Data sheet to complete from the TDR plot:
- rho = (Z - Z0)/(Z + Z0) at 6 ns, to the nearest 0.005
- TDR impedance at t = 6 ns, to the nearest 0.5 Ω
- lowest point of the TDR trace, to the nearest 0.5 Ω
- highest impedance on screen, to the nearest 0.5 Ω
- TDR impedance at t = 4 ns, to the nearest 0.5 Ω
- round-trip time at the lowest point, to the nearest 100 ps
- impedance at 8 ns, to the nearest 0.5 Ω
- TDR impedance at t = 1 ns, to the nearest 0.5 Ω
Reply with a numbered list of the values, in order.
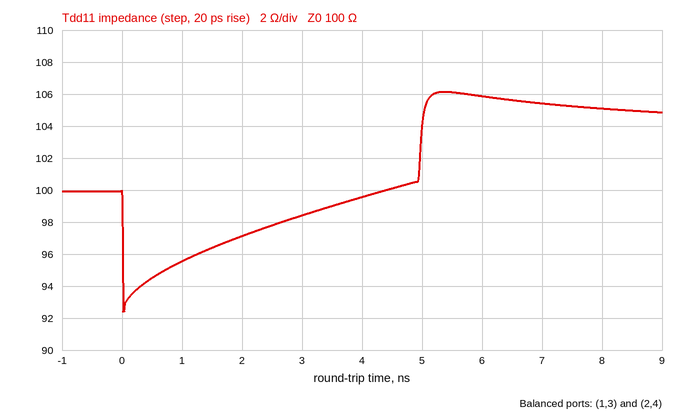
1. +0.030
2. 106.0 Ω
3. 92.5 Ω
4. 106.0 Ω
5. 99.5 Ω
6. 0.0 ns
7. 105.0 Ω
8. 95.5 Ω
